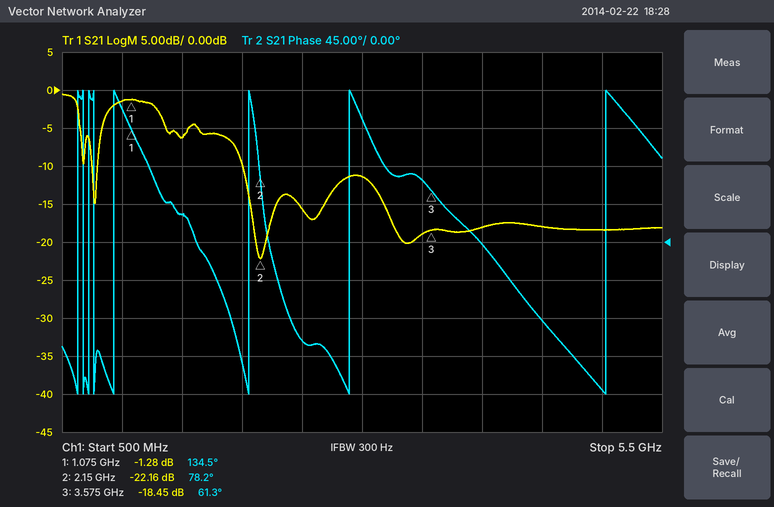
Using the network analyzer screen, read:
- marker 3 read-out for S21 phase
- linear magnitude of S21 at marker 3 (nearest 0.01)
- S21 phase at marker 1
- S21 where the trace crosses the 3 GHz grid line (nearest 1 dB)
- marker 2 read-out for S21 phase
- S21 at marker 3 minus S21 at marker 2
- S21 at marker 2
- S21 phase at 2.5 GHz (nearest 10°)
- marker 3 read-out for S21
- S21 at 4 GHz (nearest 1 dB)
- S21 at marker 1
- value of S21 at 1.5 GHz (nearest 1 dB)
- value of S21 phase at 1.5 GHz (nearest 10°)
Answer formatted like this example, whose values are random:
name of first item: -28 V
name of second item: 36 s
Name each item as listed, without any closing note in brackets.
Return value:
marker 3 read-out for S21 phase: 61.3°
linear magnitude of S21 at marker 3: 0.12
S21 phase at marker 1: 134.5°
S21 where the trace crosses the 3 GHz grid line: -11 dB
marker 2 read-out for S21 phase: 78.2°
S21 at marker 3 minus S21 at marker 2: 3.71 dB
S21 at marker 2: -22.16 dB
S21 phase at 2.5 GHz: -120°
marker 3 read-out for S21: -18.45 dB
S21 at 4 GHz: -18 dB
S21 at marker 1: -1.28 dB
value of S21 at 1.5 GHz: -6 dB
value of S21 phase at 1.5 GHz: 30°
